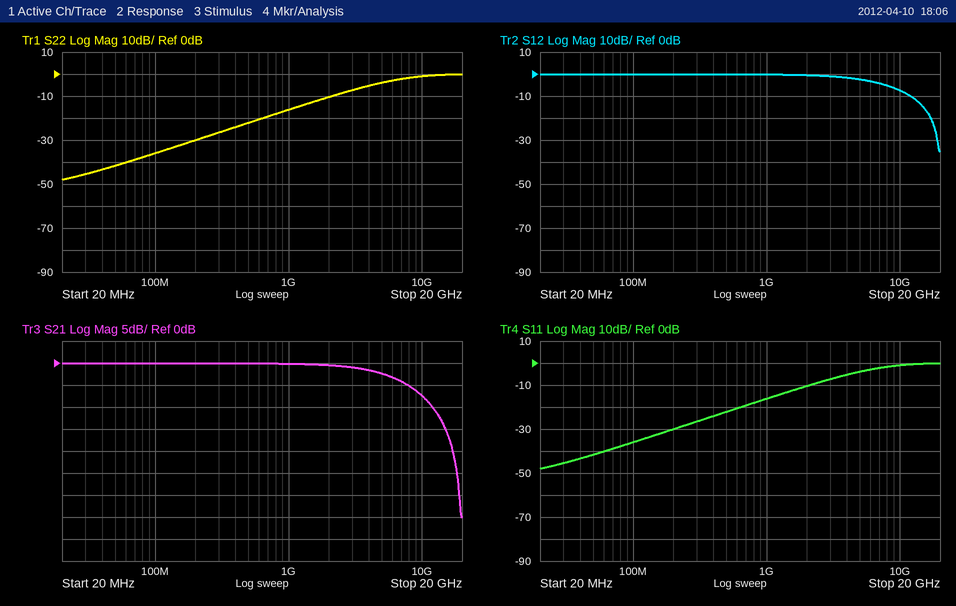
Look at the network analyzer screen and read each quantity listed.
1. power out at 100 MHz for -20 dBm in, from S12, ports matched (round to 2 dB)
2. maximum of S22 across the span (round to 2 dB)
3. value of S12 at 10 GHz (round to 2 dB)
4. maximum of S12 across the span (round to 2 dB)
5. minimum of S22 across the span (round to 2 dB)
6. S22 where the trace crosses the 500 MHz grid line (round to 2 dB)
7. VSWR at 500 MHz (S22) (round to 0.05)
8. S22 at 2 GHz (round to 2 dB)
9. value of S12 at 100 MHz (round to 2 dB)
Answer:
-20 dBm
0 dB
-8 dB
0 dB
-48 dB
-22 dB
1.15
-10 dB
0 dB
